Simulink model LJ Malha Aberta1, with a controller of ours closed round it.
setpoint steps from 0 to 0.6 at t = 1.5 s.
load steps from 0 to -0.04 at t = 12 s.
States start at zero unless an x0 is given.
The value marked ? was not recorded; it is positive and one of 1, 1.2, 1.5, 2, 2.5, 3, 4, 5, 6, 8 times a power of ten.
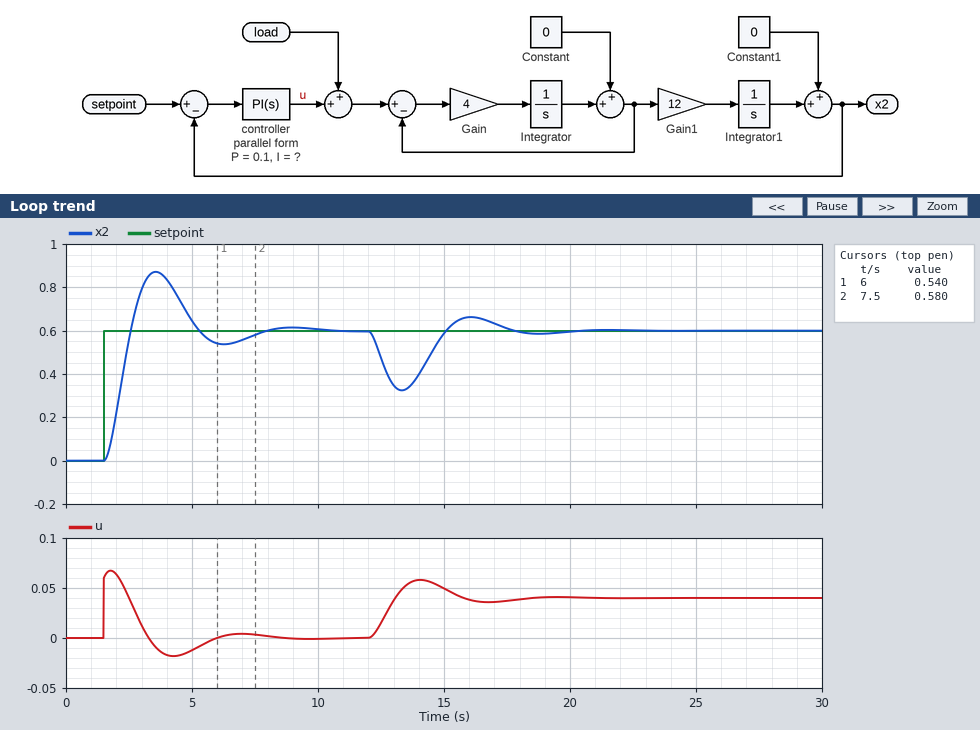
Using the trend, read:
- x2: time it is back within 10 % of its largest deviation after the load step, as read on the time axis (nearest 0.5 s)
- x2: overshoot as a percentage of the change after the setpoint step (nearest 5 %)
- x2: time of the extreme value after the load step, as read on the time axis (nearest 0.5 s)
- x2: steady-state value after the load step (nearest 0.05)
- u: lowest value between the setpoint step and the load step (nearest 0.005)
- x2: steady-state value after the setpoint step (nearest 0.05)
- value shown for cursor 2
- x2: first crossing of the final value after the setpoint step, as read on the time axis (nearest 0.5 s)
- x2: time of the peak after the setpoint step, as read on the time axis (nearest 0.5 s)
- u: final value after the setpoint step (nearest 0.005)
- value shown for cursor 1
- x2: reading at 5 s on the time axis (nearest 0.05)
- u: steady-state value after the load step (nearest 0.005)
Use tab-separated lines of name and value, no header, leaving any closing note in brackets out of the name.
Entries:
x2: time it is back within 10 % of its largest deviation after the load step, as read on the time axis	17.0 s
x2: overshoot as a percentage of the change after the setpoint step	45 %
x2: time of the extreme value after the load step, as read on the time axis	13.5 s
x2: steady-state value after the load step	0.60
u: lowest value between the setpoint step and the load step	-0.020
x2: steady-state value after the setpoint step	0.60
value shown for cursor 2	0.580
x2: first crossing of the final value after the setpoint step, as read on the time axis	2.5 s
x2: time of the peak after the setpoint step, as read on the time axis	3.5 s
u: final value after the setpoint step	0.000
value shown for cursor 1	0.540
x2: reading at 5 s on the time axis	0.65
u: steady-state value after the load step	0.040
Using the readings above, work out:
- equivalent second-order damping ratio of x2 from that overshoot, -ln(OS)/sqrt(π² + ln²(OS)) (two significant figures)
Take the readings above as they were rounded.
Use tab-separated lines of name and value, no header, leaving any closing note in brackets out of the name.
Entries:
equivalent second-order damping ratio of x2 from that overshoot, -ln(OS)/sqrt(π² + ln²(OS))	0.25
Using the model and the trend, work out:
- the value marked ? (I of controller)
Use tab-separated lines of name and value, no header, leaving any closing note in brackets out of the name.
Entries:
the value marked ?	0.1
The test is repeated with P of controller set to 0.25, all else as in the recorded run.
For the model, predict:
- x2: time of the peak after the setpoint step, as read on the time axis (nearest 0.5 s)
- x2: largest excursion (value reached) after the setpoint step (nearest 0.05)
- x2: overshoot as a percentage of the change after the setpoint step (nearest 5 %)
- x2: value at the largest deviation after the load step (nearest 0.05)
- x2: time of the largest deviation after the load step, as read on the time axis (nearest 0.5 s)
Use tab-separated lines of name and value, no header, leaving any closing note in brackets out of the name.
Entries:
x2: time of the peak after the setpoint step, as read on the time axis	2.5 s
x2: largest excursion (value reached) after the setpoint step	0.75
x2: overshoot as a percentage of the change after the setpoint step	25 %
x2: value at the largest deviation after the load step	0.45
x2: time of the largest deviation after the load step, as read on the time axis	13.0 s
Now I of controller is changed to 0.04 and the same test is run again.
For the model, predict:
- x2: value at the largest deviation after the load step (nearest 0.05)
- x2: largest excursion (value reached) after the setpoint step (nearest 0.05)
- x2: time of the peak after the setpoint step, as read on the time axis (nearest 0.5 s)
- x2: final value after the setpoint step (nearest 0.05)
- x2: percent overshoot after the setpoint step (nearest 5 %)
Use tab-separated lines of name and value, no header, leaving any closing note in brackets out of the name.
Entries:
x2: value at the largest deviation after the load step	0.30
x2: largest excursion (value reached) after the setpoint step	0.75
x2: time of the peak after the setpoint step, as read on the time axis	4.0 s
x2: final value after the setpoint step	0.60
x2: percent overshoot after the setpoint step	25 %
